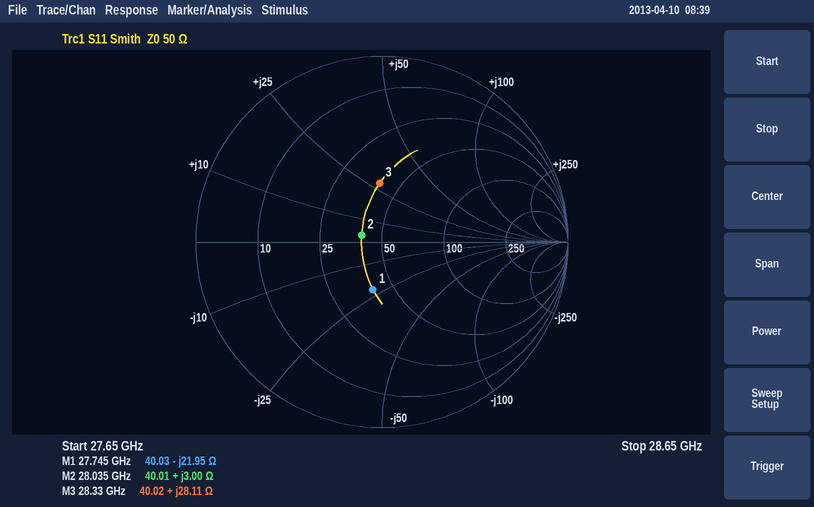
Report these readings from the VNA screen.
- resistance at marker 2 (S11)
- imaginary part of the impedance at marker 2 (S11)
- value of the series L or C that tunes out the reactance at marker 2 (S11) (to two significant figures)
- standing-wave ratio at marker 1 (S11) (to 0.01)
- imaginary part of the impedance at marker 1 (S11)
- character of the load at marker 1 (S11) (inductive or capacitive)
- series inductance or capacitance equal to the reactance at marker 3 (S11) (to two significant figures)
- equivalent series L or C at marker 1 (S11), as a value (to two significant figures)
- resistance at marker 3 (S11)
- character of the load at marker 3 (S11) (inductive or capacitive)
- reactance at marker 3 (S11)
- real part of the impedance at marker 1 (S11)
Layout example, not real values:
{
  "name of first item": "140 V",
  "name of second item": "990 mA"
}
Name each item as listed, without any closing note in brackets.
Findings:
{
  "resistance at marker 2": "40.01 Ω",
  "imaginary part of the impedance at marker 2": "+3.00 Ω",
  "value of the series L or C that tunes out the reactance at marker 2 (S11)": "1.9 pF",
  "standing-wave ratio at marker 1 (S11)": "1.70",
  "imaginary part of the impedance at marker 1": "-21.95 Ω",
  "character of the load at marker 1 (S11)": "capacitive",
  "series inductance or capacitance equal to the reactance at marker 3 (S11)": "160 pH",
  "equivalent series L or C at marker 1 (S11), as a value": "260 fF",
  "resistance at marker 3": "40.02 Ω",
  "character of the load at marker 3 (S11)": "inductive",
  "reactance at marker 3": "+28.11 Ω",
  "real part of the impedance at marker 1": "40.03 Ω"
}
